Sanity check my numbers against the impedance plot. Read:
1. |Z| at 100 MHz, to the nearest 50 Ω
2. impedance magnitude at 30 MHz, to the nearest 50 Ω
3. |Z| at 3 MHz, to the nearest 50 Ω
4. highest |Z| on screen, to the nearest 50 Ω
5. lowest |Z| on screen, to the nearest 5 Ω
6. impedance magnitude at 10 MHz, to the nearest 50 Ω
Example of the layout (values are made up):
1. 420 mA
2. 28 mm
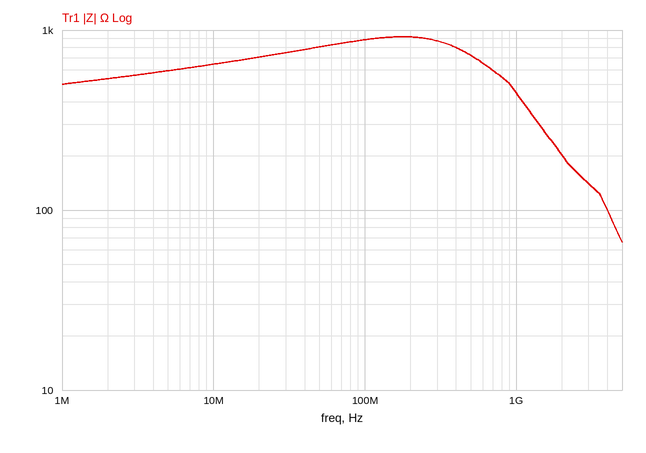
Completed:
1. 900 Ω
2. 750 Ω
3. 550 Ω
4. 900 Ω
5. 65 Ω
6. 650 Ω
